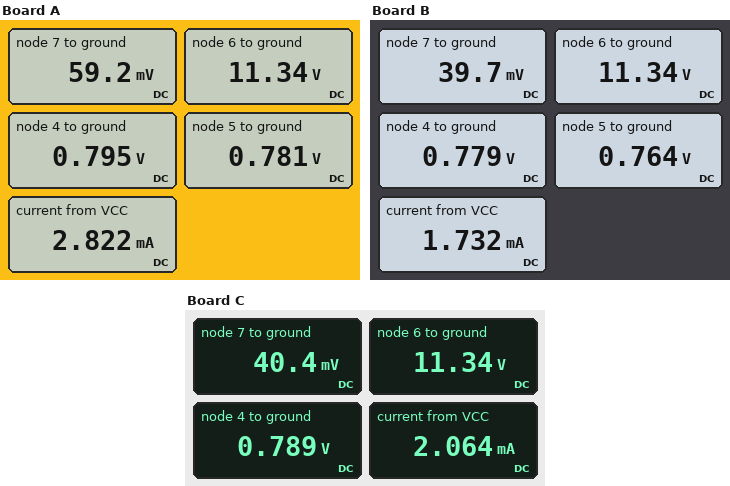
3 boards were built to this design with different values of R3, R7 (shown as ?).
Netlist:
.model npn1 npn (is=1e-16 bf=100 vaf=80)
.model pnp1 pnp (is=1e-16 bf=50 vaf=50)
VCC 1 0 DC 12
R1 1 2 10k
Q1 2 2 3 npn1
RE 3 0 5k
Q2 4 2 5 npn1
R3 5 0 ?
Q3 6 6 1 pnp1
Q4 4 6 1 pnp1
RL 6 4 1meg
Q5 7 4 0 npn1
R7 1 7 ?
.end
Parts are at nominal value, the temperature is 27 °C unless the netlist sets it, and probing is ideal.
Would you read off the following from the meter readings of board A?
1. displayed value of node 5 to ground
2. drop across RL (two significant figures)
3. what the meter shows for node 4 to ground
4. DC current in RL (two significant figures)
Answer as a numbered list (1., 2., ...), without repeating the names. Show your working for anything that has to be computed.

1. 0.781 V
2. 11.34 V - 795 mV = 11 V
3. 0.795 V
4. (11.34 V - 795 mV) / 1 MΩ = 11 µA
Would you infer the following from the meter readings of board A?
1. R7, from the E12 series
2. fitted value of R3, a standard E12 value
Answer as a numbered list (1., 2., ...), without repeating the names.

1. 6.8 kΩ
2. 1.2 kΩ
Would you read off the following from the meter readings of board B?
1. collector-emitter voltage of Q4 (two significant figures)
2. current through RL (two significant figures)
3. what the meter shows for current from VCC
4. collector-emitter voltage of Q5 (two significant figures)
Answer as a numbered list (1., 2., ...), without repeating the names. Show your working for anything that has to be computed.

1. 779 mV - 12 V = -11 V
2. (11.34 V - 779 mV) / 1 MΩ = 11 µA
3. 1.732 mA
4. 39.7 mV = 40 mV
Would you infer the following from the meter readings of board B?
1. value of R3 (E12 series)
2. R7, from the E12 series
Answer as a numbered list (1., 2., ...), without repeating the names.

1. 1.2 kΩ
2. 18 kΩ
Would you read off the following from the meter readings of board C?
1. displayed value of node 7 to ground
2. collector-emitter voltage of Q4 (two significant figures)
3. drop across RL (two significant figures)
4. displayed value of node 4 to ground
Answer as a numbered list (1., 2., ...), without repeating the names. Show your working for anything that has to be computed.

1. 40.4 mV
2. 789 mV - 12 V = -11 V
3. 11.34 V - 789 mV = 11 V
4. 0.789 V
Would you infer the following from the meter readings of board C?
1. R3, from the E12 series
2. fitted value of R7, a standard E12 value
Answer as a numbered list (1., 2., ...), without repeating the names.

1. 1.5 kΩ
2. 12 kΩ
